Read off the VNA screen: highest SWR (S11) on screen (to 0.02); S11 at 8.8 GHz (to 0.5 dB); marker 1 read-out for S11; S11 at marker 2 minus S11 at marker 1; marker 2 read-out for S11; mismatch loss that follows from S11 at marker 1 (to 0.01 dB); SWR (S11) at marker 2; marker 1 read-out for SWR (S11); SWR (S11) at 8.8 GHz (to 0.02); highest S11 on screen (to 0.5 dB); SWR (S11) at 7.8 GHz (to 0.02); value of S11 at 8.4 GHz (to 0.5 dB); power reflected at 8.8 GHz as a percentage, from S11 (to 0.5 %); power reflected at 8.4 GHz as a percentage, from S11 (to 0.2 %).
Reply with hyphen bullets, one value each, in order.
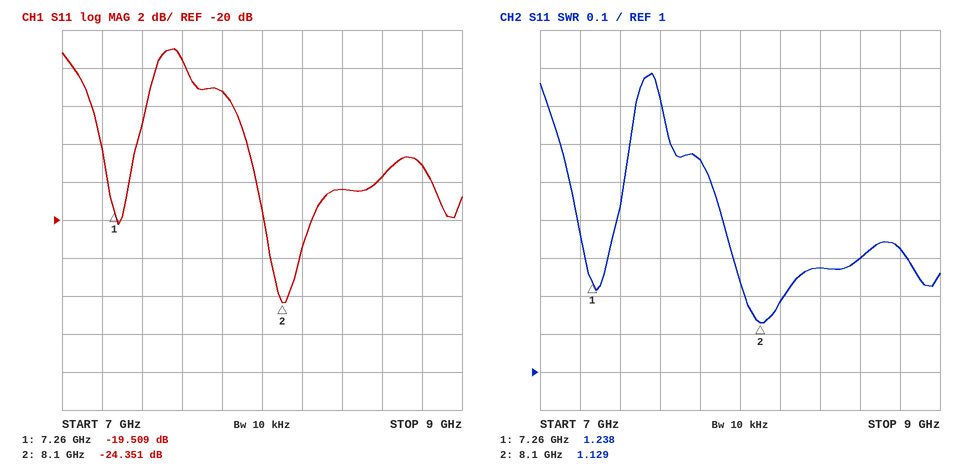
- 1.78
- -17.0 dB
- -19.509 dB
- -4.842 dB
- -24.351 dB
- 0.05 dB
- 1.129
- 1.238
- 1.32
- -11.0 dB
- 1.56
- -18.5 dB
- 2.0 %
- 1.4 %
